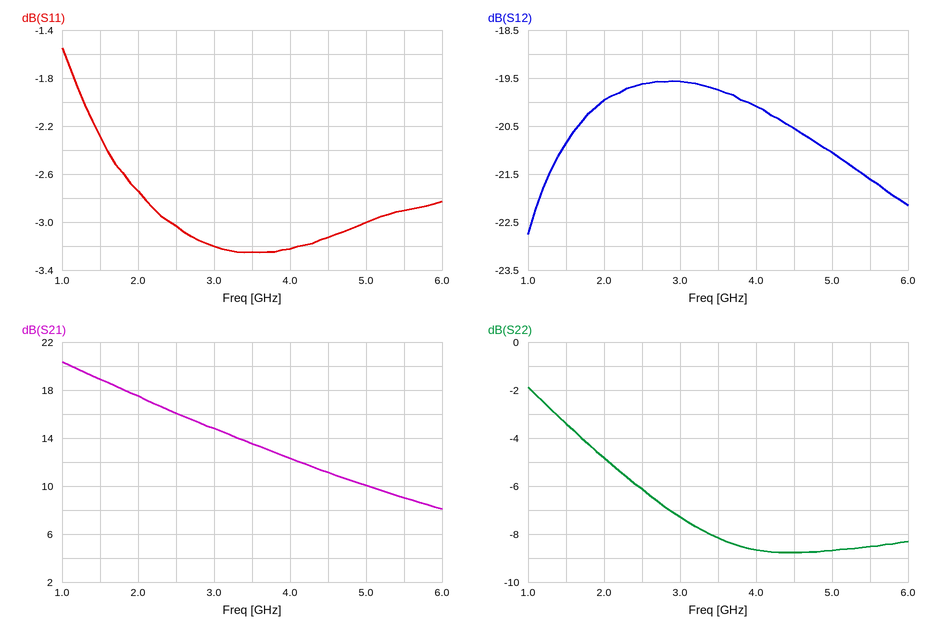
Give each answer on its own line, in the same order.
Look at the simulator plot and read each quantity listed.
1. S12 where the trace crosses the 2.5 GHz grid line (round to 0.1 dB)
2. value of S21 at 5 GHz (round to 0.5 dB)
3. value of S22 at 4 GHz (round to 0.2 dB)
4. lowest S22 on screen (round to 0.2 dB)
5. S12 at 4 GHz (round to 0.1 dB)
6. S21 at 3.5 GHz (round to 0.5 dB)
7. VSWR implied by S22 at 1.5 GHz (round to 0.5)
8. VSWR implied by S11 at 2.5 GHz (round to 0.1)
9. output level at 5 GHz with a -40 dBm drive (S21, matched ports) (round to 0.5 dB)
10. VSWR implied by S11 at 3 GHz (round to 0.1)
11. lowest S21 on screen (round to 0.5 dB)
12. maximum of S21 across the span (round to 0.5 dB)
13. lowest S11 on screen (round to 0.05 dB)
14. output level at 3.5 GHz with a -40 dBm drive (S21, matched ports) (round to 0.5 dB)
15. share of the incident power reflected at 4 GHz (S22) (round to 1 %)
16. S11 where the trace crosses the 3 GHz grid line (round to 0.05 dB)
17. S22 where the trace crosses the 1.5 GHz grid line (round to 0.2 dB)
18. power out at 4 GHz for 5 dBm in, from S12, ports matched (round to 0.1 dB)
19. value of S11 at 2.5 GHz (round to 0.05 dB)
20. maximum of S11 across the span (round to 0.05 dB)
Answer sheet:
-19.6 dB
10.0 dB
-8.6 dB
-8.8 dB
-20.1 dB
13.5 dB
5.0
5.8
-30.0 dBm
5.5
8.0 dB
20.5 dB
-3.25 dB
-26.5 dBm
14 %
-3.20 dB
-3.4 dB
-15.1 dBm
-3.05 dB
-1.55 dB
